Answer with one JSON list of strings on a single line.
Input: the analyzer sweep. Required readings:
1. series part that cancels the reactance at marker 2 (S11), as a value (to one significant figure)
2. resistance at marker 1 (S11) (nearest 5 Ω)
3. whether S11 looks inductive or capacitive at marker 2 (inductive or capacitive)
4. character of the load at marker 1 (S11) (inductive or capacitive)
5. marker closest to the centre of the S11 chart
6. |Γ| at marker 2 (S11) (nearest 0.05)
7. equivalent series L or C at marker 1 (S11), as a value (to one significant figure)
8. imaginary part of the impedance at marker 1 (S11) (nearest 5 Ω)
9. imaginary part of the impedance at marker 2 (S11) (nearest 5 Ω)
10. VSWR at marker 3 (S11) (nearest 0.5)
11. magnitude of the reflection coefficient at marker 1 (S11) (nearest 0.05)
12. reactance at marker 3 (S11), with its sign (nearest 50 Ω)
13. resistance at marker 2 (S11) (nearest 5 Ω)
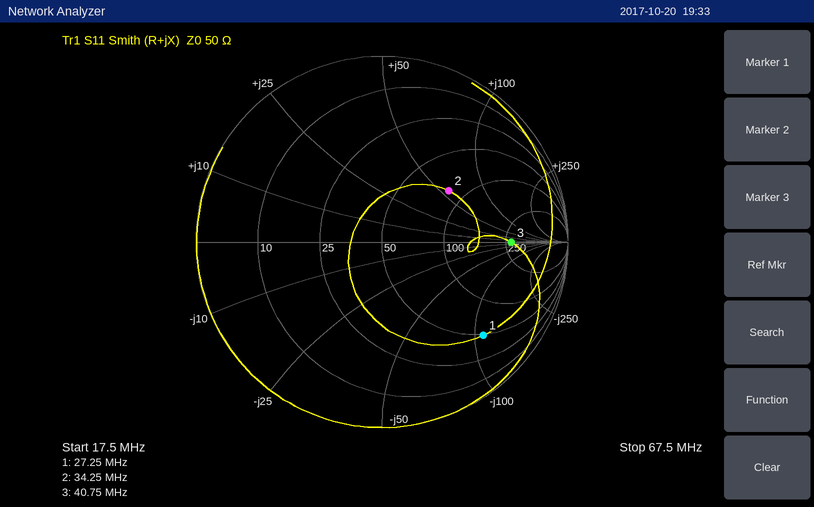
["80 pF", "50 Ω", "inductive", "capacitive", "marker 2", "0.45", "50 pF", "-110 Ω", "+55 Ω", "5.5", "0.75", "0 Ω", "80 Ω"]
